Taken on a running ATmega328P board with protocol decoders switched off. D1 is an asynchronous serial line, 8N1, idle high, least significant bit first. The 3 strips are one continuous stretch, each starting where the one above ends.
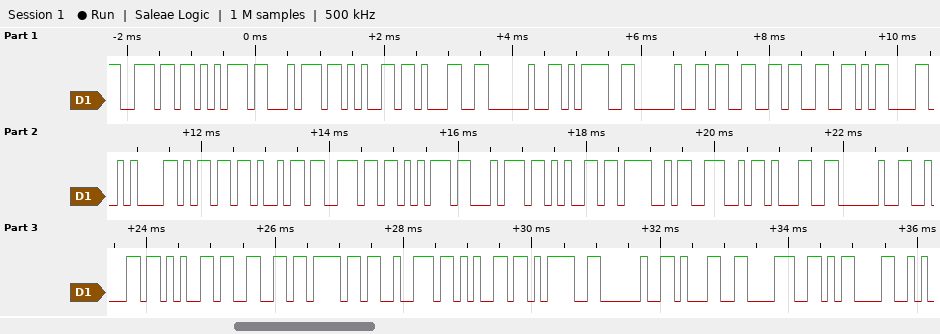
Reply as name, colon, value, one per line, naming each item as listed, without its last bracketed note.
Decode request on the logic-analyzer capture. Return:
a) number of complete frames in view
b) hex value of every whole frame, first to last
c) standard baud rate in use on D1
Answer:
number of complete frames in view: 33
hex value of every whole frame, first to last: 0x6E 0x75 0x74 0x65 0x31 0x20 0x3D 0x20 0x33 0x33 0x0D 0x0A 0x6D 0x69 0x6E 0x75 0x74 0x65 0x4F 0x4E 0x31 0x20 0x62 0x65 0x66 0x6F 0x72 0x65 0x3D 0x20 0x31 0x38 0x0D
standard baud rate in use on D1: 9600 baud
